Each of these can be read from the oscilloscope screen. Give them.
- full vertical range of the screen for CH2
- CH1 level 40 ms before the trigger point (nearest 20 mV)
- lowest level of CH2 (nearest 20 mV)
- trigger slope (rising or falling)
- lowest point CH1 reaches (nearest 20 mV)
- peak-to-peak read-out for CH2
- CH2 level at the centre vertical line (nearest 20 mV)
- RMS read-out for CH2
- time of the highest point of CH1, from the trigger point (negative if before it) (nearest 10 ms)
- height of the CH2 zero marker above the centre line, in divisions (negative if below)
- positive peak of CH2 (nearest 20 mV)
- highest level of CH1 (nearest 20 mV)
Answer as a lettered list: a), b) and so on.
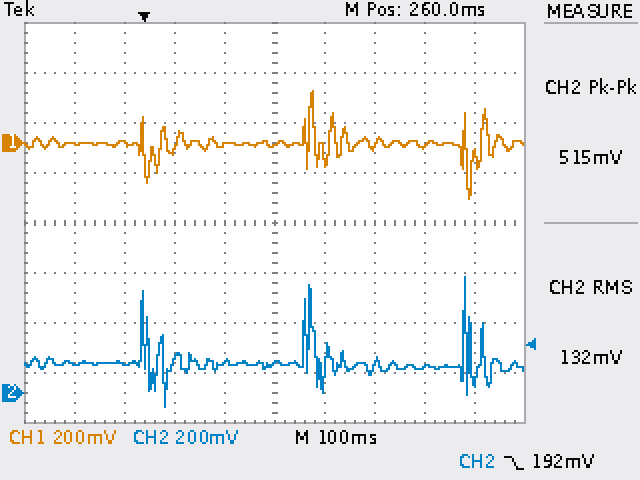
a) 1.6 V
b) 0 mV
c) -60 mV
d) falling
e) -220 mV
f) 515 mV
g) 120 mV
h) 132 mV
i) +340 ms
j) -3.4 div
k) 460 mV
l) 200 mV
